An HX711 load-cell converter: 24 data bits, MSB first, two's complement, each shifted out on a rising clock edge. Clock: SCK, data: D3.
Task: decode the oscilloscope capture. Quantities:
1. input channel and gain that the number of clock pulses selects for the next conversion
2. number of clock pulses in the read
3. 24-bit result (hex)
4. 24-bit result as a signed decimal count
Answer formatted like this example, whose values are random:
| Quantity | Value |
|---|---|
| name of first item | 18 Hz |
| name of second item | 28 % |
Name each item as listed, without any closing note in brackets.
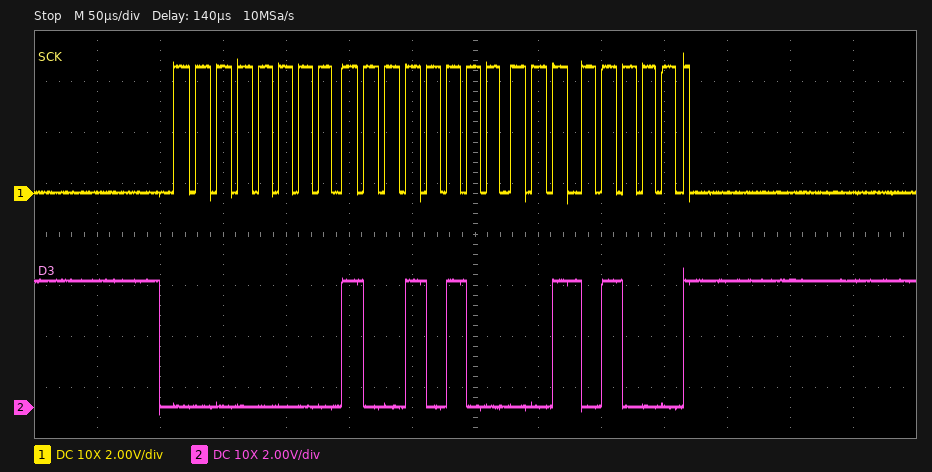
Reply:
| Quantity | Value |
|---|---|
| input channel and gain that the number of clock pulses selects for the next conversion | channel A, gain 128 |
| number of clock pulses in the read | 25 |
| 24-bit result | 0x009428 |
| 24-bit result as a signed decimal count | 37928 |
